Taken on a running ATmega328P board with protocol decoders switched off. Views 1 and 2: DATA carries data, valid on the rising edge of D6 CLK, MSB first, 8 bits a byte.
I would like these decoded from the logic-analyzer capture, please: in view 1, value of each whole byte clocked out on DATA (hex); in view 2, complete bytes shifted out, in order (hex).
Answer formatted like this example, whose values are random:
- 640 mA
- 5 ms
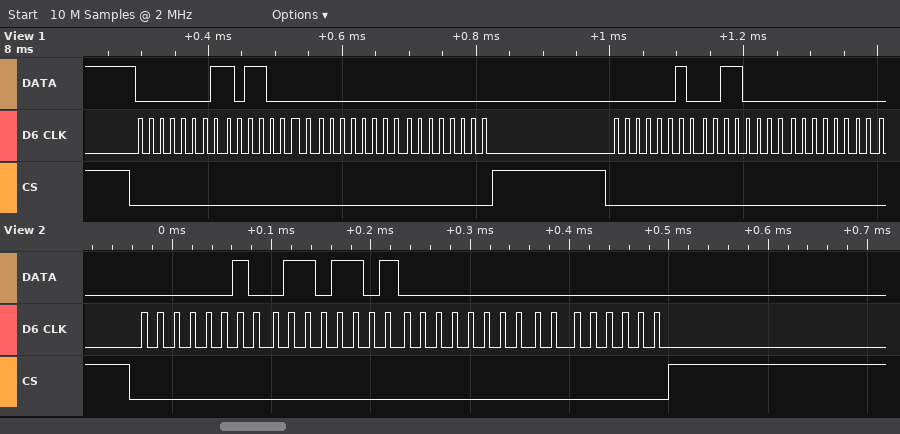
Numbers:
- 01 B0 00 00 02 30 00
- 02 6D 00 00
